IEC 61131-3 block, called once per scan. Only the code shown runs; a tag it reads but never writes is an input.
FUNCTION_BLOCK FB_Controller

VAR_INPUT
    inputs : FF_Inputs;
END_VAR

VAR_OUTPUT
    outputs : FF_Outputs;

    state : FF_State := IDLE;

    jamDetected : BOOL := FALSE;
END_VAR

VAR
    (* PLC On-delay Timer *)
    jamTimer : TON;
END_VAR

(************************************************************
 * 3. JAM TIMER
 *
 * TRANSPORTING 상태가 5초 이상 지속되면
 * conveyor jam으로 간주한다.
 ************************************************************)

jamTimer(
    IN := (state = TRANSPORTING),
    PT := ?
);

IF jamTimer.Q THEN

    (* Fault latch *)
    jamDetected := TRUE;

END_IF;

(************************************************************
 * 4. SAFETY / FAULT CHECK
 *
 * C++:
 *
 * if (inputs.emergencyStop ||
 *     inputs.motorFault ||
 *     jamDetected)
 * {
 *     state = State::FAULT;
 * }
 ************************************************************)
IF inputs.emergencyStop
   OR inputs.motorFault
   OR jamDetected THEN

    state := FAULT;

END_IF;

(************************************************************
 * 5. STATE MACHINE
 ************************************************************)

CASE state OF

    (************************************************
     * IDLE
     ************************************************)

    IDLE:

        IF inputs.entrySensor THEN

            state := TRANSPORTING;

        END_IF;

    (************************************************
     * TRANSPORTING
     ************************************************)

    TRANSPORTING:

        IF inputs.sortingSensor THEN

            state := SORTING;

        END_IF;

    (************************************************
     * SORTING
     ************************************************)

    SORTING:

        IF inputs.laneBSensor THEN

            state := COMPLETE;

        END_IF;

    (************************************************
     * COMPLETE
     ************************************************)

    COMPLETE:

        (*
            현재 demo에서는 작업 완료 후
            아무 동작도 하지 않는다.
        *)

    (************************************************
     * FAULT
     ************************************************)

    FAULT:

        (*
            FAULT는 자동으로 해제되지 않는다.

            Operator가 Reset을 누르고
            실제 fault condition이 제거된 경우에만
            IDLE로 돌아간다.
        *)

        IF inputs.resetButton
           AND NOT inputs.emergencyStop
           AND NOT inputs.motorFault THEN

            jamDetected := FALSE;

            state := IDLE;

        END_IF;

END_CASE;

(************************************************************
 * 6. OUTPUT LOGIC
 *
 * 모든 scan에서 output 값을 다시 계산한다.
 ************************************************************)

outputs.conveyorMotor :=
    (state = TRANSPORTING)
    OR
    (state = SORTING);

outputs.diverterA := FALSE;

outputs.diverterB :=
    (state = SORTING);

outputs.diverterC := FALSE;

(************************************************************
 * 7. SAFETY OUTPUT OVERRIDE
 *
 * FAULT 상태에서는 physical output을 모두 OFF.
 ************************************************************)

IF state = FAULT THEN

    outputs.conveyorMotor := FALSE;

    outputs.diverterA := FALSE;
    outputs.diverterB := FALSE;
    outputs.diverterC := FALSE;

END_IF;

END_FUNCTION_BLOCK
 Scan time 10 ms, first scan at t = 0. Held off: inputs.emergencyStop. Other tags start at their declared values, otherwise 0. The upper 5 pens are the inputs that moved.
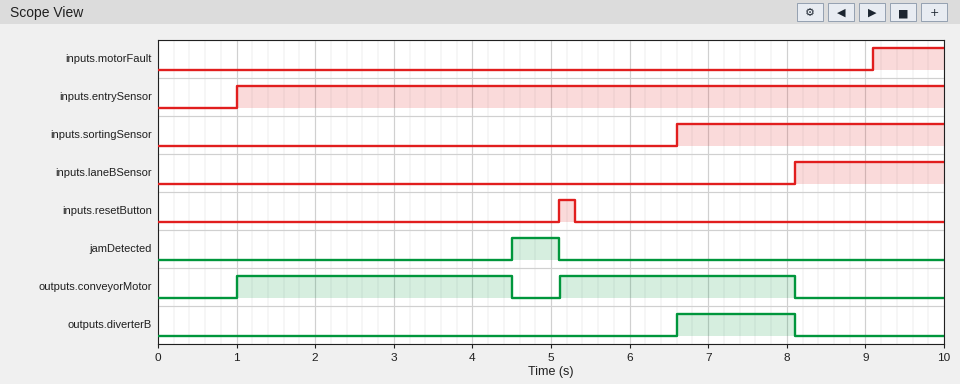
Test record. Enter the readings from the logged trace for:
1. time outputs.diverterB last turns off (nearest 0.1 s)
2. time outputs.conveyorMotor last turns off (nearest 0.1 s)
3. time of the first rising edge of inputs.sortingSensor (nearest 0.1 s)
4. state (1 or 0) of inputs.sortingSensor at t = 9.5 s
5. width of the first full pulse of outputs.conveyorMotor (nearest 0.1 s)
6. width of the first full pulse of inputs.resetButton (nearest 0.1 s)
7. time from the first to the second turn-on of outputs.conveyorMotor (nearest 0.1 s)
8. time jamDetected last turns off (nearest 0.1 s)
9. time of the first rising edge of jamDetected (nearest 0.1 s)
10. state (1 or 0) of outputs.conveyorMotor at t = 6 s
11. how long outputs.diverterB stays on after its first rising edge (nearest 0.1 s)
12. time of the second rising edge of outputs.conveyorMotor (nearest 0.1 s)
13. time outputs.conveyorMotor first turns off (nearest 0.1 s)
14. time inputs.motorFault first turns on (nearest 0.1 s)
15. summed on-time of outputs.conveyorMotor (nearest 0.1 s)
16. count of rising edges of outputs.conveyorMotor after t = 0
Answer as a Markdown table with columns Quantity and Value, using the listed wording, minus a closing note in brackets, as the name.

| Quantity | Value |
|---|---|
| time outputs.diverterB last turns off | 8.1 s |
| time outputs.conveyorMotor last turns off | 8.1 s |
| time of the first rising edge of inputs.sortingSensor | 6.6 s |
| state (1 or 0) of inputs.sortingSensor at t = 9.5 s | 1 |
| width of the first full pulse of outputs.conveyorMotor | 3.5 s |
| width of the first full pulse of inputs.resetButton | 0.2 s |
| time from the first to the second turn-on of outputs.conveyorMotor | 4.1 s |
| time jamDetected last turns off | 5.1 s |
| time of the first rising edge of jamDetected | 4.5 s |
| state (1 or 0) of outputs.conveyorMotor at t = 6 s | 1 |
| how long outputs.diverterB stays on after its first rising edge | 1.5 s |
| time of the second rising edge of outputs.conveyorMotor | 5.1 s |
| time outputs.conveyorMotor first turns off | 4.5 s |
| time inputs.motorFault first turns on | 9.1 s |
| summed on-time of outputs.conveyorMotor | 6.5 s |
| count of rising edges of outputs.conveyorMotor after t = 0 | 2 |
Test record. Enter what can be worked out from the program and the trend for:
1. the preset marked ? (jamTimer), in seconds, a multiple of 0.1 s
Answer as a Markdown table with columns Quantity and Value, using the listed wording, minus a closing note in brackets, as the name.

| Quantity | Value |
|---|---|
| the preset marked ? (jamTimer), in seconds, a multiple of 0.1 s | 3.5 s |
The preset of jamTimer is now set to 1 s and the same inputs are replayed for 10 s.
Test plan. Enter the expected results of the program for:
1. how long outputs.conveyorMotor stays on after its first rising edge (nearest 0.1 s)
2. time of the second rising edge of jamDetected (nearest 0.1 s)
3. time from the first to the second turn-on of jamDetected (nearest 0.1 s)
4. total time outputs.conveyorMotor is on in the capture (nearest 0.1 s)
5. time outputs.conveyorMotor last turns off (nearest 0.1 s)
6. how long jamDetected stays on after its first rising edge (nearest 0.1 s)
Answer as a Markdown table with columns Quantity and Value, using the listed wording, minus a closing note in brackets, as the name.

| Quantity | Value |
|---|---|
| how long outputs.conveyorMotor stays on after its first rising edge | 1.0 s |
| time of the second rising edge of jamDetected | 6.1 s |
| time from the first to the second turn-on of jamDetected | 4.1 s |
| total time outputs.conveyorMotor is on in the capture | 2.0 s |
| time outputs.conveyorMotor last turns off | 6.1 s |
| how long jamDetected stays on after its first rising edge | 3.1 s |
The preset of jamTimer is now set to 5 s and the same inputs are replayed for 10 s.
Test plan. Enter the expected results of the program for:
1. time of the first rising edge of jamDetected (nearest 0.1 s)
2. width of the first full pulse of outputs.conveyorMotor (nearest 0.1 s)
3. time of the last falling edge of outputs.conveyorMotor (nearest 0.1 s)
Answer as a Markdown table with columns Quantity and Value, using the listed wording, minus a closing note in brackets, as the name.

| Quantity | Value |
|---|---|
| time of the first rising edge of jamDetected | 6.0 s |
| width of the first full pulse of outputs.conveyorMotor | 5.0 s |
| time of the last falling edge of outputs.conveyorMotor | 6.0 s |
